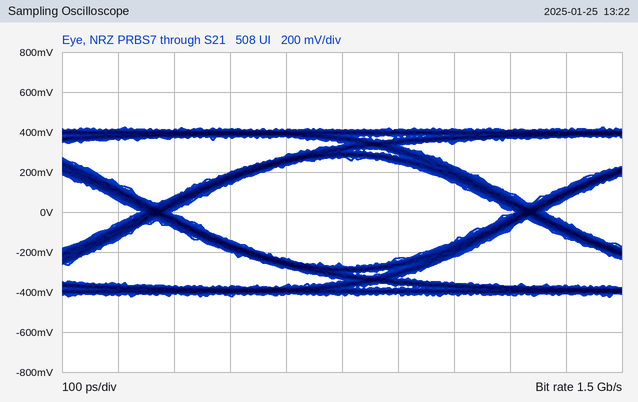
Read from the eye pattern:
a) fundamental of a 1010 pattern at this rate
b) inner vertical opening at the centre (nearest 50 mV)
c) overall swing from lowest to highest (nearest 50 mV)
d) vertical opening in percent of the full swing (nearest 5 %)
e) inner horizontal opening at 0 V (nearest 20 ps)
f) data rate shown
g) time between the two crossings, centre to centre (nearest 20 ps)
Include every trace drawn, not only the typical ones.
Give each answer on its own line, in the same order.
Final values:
750 MHz
550 mV
850 mV
65 %
620 ps
1.5 Gb/s
660 ps
